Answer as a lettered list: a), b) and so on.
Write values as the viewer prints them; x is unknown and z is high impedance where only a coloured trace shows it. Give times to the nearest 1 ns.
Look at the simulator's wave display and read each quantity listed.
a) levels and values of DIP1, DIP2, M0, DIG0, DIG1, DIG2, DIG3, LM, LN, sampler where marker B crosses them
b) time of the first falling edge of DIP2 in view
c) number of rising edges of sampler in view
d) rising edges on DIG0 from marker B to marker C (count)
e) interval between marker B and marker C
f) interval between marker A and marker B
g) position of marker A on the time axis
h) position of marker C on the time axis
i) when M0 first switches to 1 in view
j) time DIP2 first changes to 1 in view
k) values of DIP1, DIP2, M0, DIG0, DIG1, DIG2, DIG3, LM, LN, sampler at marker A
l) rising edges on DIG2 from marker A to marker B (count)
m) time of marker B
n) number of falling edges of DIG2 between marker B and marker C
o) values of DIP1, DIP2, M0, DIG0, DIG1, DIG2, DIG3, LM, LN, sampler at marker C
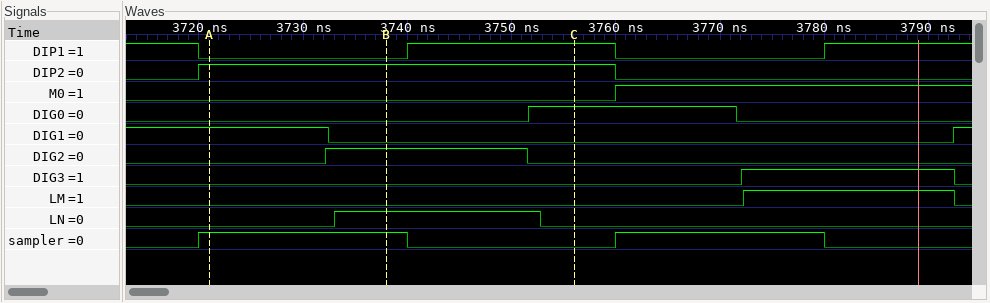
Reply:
a) DIP1=0, DIP2=1, M0=0, DIG0=0, DIG1=0, DIG2=1, DIG3=0, LM=0, LN=1, sampler=1
b) 3760 ns
c) 2
d) 1
e) 18 ns
f) 17 ns
g) 3721 ns
h) 3756 ns
i) 3760 ns
j) 3720 ns
k) DIP1=0, DIP2=1, M0=0, DIG0=0, DIG1=1, DIG2=0, DIG3=0, LM=0, LN=0, sampler=1
l) 1
m) 3738 ns
n) 1
o) DIP1=1, DIP2=1, M0=0, DIG0=1, DIG1=0, DIG2=0, DIG3=0, LM=0, LN=0, sampler=0
